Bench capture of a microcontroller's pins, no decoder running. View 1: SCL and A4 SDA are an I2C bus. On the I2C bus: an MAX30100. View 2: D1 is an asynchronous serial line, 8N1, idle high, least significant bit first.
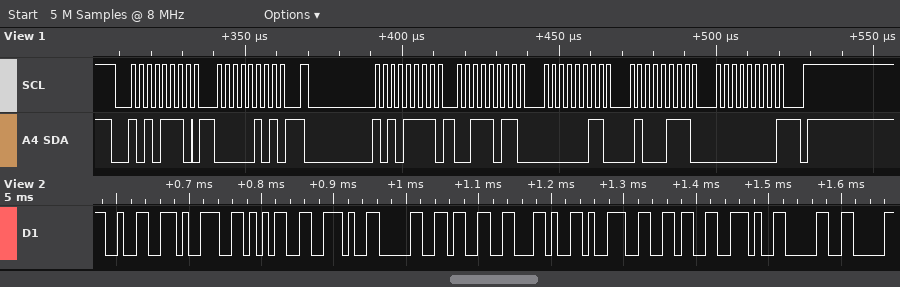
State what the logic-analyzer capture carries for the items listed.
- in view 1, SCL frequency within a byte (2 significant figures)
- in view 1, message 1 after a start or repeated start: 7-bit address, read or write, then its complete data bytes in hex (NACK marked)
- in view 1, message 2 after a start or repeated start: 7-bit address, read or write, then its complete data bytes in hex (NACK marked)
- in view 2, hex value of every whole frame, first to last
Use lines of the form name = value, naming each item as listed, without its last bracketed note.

in view 1, SCL frequency within a byte = 400 kHz
in view 1, message 1 after a start or repeated start: 7-bit address, read or write, then its complete data bytes in hex = 0x57 write: 05
in view 1, message 2 after a start or repeated start: 7-bit address, read or write, then its complete data bytes in hex = 0x57 read: 3B 03 47 00 NACK
in view 2, hex value of every whole frame, first to last = 32 39 35 2E 30 33 2C 39 36 2E 30
